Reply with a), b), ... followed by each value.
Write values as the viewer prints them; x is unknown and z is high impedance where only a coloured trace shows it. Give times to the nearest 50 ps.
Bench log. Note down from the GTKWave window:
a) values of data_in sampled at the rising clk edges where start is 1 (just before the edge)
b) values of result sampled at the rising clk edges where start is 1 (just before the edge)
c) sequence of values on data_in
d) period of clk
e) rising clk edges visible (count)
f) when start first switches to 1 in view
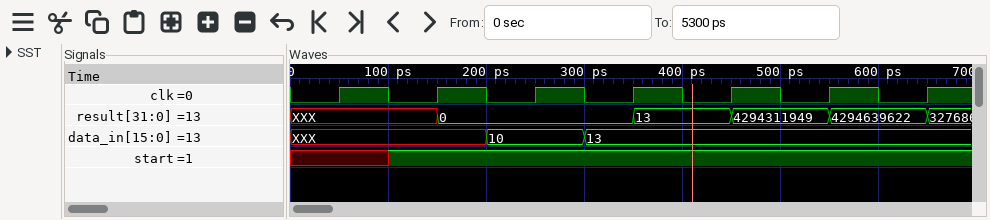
a) XXX, 10, 13, 13, 13, 13
b) XXX, 0, 0, 13, 4294311949, 4294639622
c) XXX, 10, 13
d) 100 ps
e) 7
f) 100 ps
